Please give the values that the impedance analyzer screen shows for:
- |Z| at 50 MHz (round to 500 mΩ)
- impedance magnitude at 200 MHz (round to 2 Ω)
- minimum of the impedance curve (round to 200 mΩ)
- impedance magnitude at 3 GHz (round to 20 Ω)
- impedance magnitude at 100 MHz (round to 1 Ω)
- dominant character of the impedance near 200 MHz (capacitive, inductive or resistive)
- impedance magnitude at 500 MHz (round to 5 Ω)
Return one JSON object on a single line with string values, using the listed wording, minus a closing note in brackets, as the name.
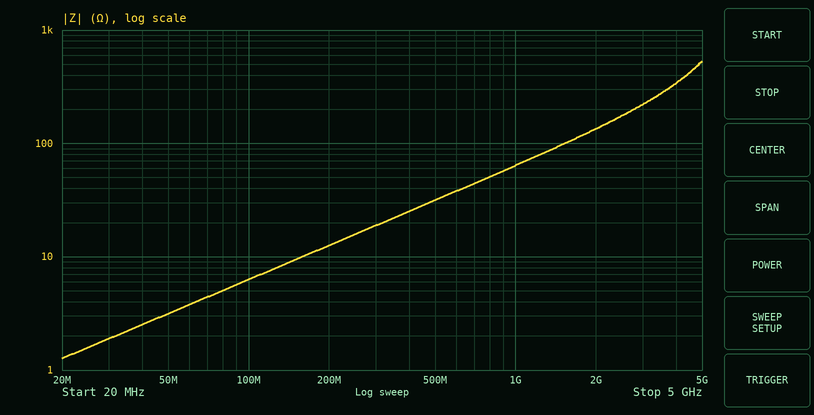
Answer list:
{"|Z| at 50 MHz": "3.0 Ω", "impedance magnitude at 200 MHz": "12 Ω", "minimum of the impedance curve": "1.2 Ω", "impedance magnitude at 3 GHz": "220 Ω", "impedance magnitude at 100 MHz": "6 Ω", "dominant character of the impedance near 200 MHz": "inductive", "impedance magnitude at 500 MHz": "30 Ω"}
